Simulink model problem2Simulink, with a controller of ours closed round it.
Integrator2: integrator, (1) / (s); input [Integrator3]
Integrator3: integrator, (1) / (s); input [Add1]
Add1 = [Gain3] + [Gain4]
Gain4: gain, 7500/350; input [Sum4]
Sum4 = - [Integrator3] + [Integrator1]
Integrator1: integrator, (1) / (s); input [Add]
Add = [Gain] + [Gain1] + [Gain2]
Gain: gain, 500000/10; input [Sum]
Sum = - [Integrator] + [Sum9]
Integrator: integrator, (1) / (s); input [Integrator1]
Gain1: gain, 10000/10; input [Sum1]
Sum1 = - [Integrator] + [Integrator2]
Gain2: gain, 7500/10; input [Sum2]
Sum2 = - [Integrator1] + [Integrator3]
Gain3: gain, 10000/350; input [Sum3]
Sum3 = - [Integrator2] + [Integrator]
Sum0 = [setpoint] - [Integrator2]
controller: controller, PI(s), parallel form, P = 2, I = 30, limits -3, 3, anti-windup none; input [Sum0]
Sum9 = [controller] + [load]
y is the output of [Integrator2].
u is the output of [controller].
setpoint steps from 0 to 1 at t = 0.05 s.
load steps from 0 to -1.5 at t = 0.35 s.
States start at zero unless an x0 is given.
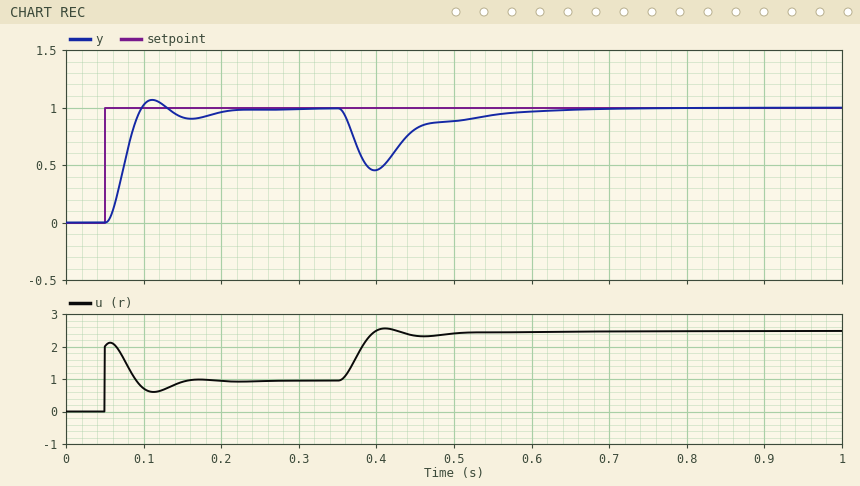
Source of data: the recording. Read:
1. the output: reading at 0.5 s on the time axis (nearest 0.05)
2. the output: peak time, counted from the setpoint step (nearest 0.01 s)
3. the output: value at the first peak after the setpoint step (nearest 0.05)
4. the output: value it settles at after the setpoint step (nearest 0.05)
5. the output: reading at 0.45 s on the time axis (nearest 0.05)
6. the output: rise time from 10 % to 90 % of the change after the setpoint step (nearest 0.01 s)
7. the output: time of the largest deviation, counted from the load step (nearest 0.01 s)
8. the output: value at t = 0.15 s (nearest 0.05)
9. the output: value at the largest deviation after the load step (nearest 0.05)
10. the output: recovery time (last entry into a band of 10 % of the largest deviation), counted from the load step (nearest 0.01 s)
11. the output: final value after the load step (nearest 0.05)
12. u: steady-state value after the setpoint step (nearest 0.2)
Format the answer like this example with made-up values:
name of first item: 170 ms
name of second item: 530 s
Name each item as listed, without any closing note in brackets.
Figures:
the output: reading at 0.5 s on the time axis: 0.90
the output: peak time, counted from the setpoint step: 0.06 s
the output: value at the first peak after the setpoint step: 1.05
the output: value it settles at after the setpoint step: 1.00
the output: reading at 0.45 s on the time axis: 0.80
the output: rise time from 10 % to 90 % of the change after the setpoint step: 0.03 s
the output: time of the largest deviation, counted from the load step: 0.05 s
the output: value at t = 0.15 s: 0.90
the output: value at the largest deviation after the load step: 0.45
the output: recovery time (last entry into a band of 10 % of the largest deviation), counted from the load step: 0.21 s
the output: final value after the load step: 1.00
u: steady-state value after the setpoint step: 1.0
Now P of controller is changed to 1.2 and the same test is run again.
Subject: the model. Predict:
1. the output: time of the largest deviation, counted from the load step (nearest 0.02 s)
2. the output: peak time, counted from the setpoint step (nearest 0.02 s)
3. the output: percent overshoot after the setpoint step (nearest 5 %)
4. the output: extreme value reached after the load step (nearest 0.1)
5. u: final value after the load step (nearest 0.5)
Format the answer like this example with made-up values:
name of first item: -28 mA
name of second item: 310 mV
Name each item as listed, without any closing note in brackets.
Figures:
the output: time of the largest deviation, counted from the load step: 0.06 s
the output: peak time, counted from the setpoint step: 0.08 s
the output: percent overshoot after the setpoint step: 10 %
the output: extreme value reached after the load step: 0.3
u: final value after the load step: 2.5
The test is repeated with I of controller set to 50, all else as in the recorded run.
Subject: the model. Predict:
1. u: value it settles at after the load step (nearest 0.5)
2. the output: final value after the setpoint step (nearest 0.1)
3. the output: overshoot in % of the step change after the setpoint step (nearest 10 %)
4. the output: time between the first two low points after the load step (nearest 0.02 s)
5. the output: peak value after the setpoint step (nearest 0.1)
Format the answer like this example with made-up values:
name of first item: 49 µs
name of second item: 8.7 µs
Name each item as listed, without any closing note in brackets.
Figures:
u: value it settles at after the load step: 2.5
the output: final value after the setpoint step: 1.0
the output: overshoot in % of the step change after the setpoint step: 20 %
the output: time between the first two low points after the load step: 0.12 s
the output: peak value after the setpoint step: 1.2
